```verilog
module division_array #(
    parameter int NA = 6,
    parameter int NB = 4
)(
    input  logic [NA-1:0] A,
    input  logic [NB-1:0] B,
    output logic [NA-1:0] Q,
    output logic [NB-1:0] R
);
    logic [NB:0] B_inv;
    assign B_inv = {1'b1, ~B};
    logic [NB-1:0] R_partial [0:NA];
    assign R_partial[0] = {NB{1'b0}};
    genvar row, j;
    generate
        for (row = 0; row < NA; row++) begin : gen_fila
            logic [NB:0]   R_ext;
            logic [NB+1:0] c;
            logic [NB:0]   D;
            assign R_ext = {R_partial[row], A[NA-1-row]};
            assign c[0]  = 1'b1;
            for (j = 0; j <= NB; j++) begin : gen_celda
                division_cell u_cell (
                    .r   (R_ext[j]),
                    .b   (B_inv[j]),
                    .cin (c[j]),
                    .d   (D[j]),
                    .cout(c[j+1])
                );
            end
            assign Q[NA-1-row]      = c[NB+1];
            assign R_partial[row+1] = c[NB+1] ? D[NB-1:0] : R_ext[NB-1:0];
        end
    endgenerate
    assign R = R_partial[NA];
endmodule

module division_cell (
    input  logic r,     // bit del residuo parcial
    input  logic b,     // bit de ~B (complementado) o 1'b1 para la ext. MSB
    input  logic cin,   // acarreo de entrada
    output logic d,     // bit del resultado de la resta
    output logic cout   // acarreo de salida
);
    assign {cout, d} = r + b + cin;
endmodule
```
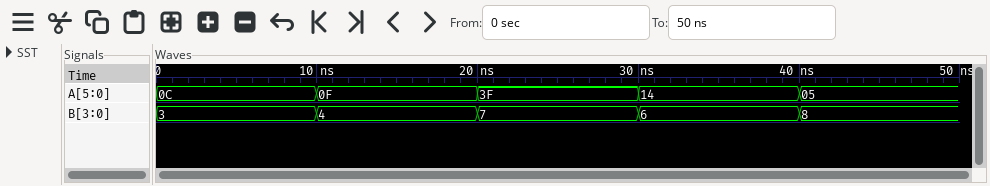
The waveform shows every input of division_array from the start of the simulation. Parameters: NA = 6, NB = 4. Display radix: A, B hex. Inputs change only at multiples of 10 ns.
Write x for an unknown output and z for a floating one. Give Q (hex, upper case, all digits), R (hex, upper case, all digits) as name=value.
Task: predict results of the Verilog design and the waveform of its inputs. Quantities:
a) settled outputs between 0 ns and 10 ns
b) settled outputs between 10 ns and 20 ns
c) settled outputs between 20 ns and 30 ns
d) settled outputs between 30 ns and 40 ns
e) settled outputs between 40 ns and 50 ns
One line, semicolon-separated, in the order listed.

Q=04, R=0; Q=03, R=3; Q=09, R=0; Q=03, R=2; Q=00, R=5
